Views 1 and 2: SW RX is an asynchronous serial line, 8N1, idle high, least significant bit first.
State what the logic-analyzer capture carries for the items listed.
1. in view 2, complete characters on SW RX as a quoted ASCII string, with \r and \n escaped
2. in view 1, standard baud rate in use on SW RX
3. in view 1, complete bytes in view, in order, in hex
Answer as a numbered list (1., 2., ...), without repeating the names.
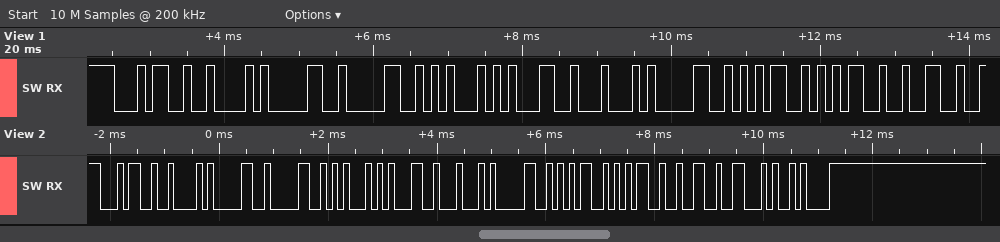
1. "4B00E1D0552F\n"
2. 9600 baud
3. 34 42 30 30 45 31 44 30 35 35 32
